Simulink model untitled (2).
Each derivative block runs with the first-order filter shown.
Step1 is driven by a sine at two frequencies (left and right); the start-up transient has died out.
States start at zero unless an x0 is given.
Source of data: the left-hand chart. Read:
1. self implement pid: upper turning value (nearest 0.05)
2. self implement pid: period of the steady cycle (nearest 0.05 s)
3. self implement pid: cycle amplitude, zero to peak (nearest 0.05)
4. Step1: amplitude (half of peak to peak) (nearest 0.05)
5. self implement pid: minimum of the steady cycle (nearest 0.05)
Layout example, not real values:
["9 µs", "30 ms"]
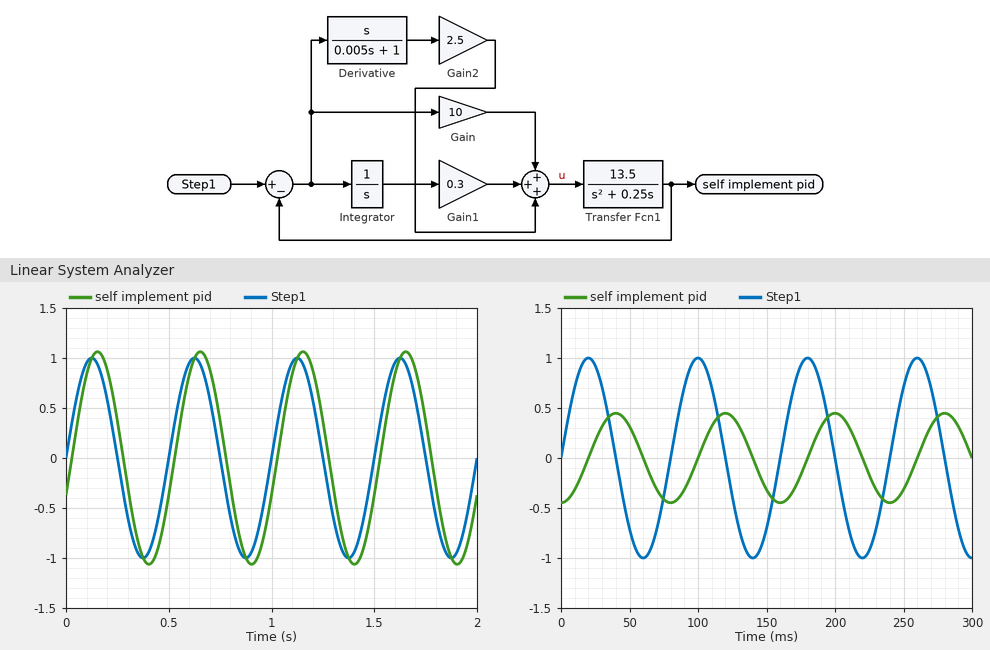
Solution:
["1.05", "0.50 s", "1.05", "1.00", "-1.05"]
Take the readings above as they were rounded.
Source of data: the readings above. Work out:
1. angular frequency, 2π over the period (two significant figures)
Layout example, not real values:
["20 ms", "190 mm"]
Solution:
["13 rad/s"]
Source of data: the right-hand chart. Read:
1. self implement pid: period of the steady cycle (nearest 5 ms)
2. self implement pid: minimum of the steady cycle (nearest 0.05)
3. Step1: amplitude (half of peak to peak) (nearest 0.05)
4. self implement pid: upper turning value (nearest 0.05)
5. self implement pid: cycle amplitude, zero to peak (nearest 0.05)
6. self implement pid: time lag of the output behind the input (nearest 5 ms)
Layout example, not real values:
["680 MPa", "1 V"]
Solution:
["80 ms", "-0.45", "1.00", "0.45", "0.45", "20 ms"]
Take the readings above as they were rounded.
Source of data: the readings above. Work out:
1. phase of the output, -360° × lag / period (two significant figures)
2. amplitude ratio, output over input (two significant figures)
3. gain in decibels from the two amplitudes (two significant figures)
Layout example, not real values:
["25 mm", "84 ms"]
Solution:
["-90°", "0.45", "-6.9 dB"]
